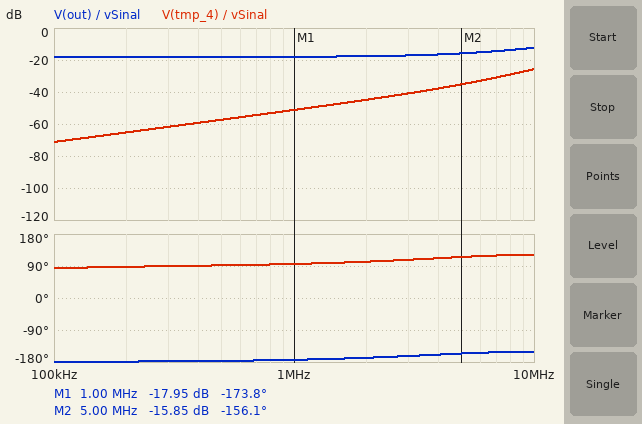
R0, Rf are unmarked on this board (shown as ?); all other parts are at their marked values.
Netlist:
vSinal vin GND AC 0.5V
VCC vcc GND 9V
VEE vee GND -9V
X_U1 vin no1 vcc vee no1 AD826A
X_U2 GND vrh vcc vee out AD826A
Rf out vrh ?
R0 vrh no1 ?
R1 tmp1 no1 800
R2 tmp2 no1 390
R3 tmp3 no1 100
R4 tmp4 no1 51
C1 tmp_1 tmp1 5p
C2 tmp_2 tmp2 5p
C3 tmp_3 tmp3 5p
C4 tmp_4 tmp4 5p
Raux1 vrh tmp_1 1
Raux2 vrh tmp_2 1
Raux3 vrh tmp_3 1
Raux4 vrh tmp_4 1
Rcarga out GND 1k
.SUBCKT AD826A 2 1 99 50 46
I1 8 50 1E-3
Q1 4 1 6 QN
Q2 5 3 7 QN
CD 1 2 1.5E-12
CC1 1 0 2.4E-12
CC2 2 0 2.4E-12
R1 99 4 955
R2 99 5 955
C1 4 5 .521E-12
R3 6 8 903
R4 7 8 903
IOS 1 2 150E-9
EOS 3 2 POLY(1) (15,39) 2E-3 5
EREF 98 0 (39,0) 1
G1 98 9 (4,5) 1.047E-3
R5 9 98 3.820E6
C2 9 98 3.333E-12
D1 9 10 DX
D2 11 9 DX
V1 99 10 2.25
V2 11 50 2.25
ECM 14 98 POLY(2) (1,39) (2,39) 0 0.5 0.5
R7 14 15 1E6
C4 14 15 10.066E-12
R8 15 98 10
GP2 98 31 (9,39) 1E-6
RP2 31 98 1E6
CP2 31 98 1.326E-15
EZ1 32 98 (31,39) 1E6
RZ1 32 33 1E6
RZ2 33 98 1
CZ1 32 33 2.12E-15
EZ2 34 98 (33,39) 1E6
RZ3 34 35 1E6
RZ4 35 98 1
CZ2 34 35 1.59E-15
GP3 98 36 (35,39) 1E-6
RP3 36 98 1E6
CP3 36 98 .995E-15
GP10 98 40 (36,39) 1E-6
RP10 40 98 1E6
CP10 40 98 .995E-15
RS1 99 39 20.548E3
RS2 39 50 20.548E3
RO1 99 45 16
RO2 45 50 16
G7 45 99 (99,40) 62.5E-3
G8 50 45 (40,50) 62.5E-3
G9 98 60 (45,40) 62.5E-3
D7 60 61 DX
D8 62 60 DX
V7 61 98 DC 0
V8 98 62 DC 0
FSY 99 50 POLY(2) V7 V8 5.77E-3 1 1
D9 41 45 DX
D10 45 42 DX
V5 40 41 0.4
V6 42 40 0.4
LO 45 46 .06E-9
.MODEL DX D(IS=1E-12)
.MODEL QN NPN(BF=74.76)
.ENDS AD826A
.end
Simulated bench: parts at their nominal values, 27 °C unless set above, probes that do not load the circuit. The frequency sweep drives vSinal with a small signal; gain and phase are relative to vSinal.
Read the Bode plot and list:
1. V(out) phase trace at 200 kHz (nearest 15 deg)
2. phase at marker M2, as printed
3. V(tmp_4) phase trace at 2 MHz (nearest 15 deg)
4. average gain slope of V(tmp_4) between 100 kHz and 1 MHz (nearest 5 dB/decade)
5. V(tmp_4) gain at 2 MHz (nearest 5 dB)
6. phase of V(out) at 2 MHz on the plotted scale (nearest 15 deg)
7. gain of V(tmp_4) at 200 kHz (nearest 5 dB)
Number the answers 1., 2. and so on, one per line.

1. -180 deg
2. -156.1 deg
3. 105 deg
4. 20 dB/decade
5. -45 dB
6. -165 deg
7. -65 dB
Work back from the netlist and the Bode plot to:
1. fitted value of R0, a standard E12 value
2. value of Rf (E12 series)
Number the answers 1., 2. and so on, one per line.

1. 1.2 kΩ
2. 150 Ω
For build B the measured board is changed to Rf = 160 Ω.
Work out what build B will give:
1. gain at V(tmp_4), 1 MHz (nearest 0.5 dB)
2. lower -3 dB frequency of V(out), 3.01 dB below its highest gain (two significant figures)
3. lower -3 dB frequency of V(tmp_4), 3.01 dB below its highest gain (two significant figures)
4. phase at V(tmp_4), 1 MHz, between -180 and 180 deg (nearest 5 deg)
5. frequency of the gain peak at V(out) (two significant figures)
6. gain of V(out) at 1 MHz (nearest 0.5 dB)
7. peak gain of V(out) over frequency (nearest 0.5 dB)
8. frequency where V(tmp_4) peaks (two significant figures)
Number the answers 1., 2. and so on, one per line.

1. -50.5 dB
2. 24 MHz
3. 35 MHz
4. 95 deg
5. 42 MHz
6. -17.5 dB
7. -2.0 dB
8. 57 MHz
